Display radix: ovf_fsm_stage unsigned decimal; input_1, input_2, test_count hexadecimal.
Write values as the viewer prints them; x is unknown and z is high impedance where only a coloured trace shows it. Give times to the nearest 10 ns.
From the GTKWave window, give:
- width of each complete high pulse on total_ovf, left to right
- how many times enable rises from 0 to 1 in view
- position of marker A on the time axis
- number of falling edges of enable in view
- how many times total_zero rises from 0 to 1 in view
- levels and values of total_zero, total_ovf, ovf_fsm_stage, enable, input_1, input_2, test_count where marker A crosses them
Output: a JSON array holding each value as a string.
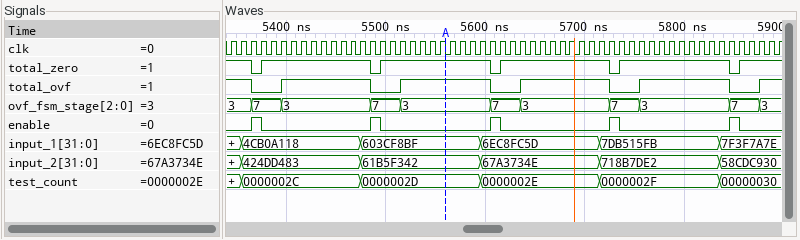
["90 ns, 90 ns, 90 ns, 90 ns", "5", "5560 ns", "5", "5", "total_zero=1, total_ovf=1, ovf_fsm_stage=3, enable=0, input_1=603CF8BF, input_2=61B5F342, test_count=0000002D"]
